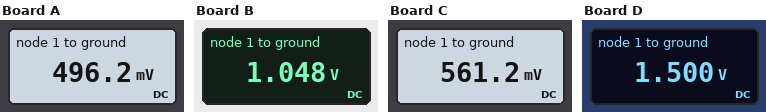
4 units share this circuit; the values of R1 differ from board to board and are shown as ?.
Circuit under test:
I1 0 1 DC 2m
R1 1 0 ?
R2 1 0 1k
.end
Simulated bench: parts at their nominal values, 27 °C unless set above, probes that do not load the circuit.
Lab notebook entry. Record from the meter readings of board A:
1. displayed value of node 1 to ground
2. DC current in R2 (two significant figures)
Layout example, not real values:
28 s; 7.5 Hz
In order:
496.2 mV; 500 µA
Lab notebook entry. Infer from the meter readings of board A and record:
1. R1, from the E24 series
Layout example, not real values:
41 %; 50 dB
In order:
330 Ω
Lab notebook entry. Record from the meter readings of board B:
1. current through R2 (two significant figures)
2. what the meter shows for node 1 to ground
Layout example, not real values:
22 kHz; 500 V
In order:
1.0 mA; 1.048 V
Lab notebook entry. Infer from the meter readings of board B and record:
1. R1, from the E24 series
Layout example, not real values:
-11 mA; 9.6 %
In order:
1.1 kΩ
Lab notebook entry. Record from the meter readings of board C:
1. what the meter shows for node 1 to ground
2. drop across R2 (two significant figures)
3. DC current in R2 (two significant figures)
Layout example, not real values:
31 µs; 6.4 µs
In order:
561.2 mV; 560 mV; 560 µA
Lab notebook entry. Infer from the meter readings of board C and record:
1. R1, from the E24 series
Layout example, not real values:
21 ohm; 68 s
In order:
390 Ω
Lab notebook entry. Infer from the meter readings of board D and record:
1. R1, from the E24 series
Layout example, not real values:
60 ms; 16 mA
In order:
3 kΩ
